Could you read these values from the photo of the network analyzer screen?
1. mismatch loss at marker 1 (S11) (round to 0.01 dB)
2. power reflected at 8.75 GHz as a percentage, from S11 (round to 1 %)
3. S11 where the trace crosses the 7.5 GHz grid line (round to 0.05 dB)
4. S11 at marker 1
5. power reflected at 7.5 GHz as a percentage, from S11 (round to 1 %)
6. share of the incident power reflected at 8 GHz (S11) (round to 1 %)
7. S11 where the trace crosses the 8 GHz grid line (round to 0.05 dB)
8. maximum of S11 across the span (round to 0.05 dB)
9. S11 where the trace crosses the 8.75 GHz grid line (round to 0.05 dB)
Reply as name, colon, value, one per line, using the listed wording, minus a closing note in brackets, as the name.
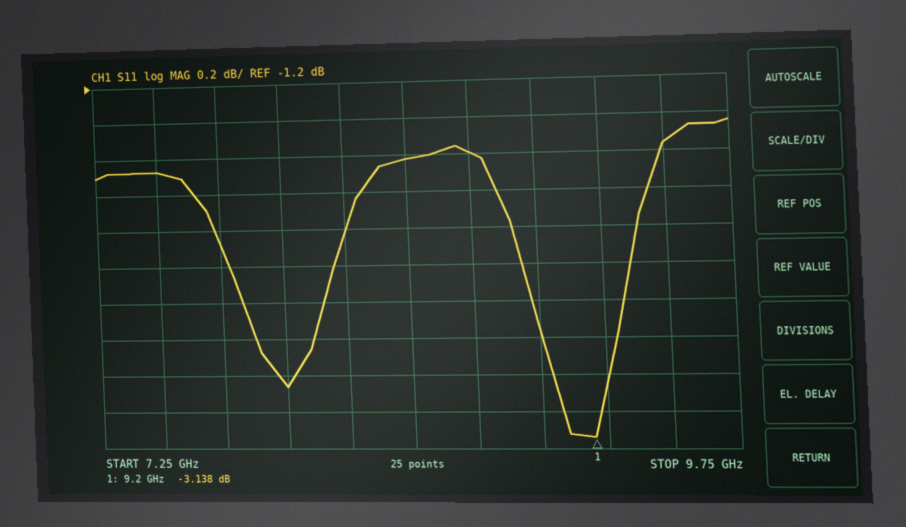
mismatch loss at marker 1 (S11): 2.89 dB
power reflected at 8.75 GHz as a percentage, from S11: 69 %
S11 where the trace crosses the 7.5 GHz grid line: -1.65 dB
S11 at marker 1: -3.138 dB
power reflected at 7.5 GHz as a percentage, from S11: 68 %
share of the incident power reflected at 8 GHz (S11): 52 %
S11 where the trace crosses the 8 GHz grid line: -2.85 dB
maximum of S11 across the span: -1.45 dB
S11 where the trace crosses the 8.75 GHz grid line: -1.60 dB
